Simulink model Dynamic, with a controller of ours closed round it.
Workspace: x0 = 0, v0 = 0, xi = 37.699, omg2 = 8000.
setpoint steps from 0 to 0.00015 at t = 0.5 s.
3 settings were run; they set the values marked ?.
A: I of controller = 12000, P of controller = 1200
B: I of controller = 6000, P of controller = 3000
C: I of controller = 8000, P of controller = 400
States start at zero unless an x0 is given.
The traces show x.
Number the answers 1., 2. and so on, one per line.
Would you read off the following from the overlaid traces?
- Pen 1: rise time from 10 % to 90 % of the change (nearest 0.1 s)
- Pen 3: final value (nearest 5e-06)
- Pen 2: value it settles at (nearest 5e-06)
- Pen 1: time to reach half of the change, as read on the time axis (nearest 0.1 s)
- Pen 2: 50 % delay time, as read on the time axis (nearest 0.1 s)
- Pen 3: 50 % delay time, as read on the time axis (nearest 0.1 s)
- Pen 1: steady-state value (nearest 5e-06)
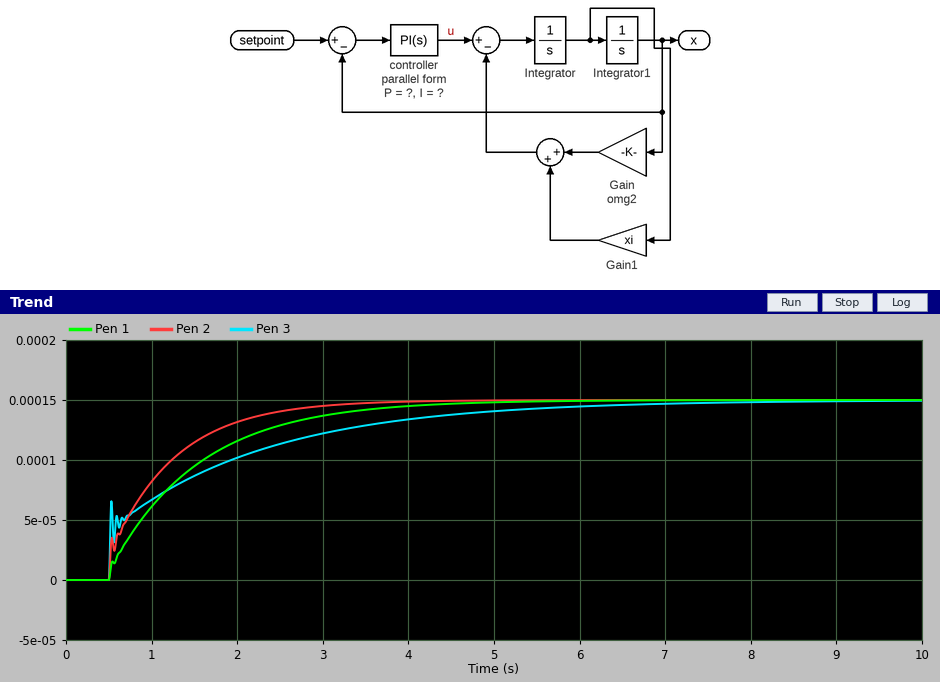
1. 2.3 s
2. 0.000150
3. 0.000150
4. 1.2 s
5. 0.9 s
6. 1.2 s
7. 0.000150
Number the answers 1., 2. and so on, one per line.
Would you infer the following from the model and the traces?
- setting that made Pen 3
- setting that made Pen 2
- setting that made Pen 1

1. B
2. A
3. C
